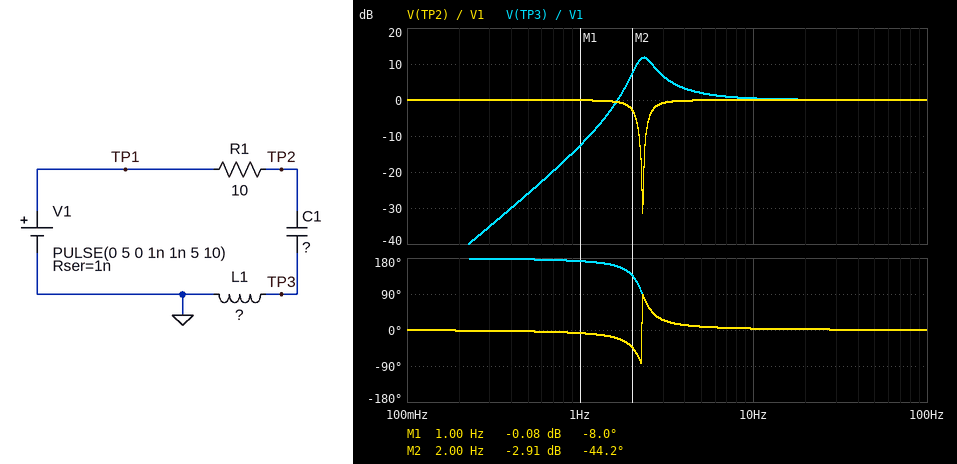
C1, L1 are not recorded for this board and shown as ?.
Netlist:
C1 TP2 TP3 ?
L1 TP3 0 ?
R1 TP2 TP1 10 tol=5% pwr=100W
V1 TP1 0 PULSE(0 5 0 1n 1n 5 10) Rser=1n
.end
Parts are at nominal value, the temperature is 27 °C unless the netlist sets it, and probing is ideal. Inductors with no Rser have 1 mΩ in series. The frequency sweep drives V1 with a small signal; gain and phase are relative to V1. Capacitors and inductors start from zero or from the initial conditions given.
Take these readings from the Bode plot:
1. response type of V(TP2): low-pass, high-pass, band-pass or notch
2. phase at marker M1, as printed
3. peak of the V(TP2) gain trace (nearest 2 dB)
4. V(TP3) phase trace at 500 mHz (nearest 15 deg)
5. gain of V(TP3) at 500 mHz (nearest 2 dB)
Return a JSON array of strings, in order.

["notch", "-8.0 deg", "0 dB", "180 deg", "-26 dB"]
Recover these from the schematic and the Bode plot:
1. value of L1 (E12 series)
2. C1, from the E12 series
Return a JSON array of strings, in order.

["2.7 H", "1.8 mF"]
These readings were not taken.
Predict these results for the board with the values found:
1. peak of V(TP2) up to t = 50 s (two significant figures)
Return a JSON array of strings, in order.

["5.7 V"]
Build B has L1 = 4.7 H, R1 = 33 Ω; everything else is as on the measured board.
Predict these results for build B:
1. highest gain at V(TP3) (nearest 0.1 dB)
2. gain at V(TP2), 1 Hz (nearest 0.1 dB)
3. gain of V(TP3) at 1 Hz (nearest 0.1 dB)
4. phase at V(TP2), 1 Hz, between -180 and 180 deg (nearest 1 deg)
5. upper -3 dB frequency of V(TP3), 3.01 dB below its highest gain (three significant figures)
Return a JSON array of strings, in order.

["4.3 dB", "-1.2 dB", "-7.2 dB", "-29 deg", "4.08 Hz"]
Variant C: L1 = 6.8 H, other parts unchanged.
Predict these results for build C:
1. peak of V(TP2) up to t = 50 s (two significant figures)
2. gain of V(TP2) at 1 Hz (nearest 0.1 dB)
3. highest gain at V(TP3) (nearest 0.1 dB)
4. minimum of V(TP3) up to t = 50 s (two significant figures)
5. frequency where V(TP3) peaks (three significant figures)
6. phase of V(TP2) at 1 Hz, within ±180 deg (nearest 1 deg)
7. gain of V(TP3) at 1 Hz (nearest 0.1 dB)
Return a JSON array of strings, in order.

["5.6 V", "-0.2 dB", "15.8 dB", "-4.9 V", "1.45 Hz", "-12 deg", "-0.8 dB"]
